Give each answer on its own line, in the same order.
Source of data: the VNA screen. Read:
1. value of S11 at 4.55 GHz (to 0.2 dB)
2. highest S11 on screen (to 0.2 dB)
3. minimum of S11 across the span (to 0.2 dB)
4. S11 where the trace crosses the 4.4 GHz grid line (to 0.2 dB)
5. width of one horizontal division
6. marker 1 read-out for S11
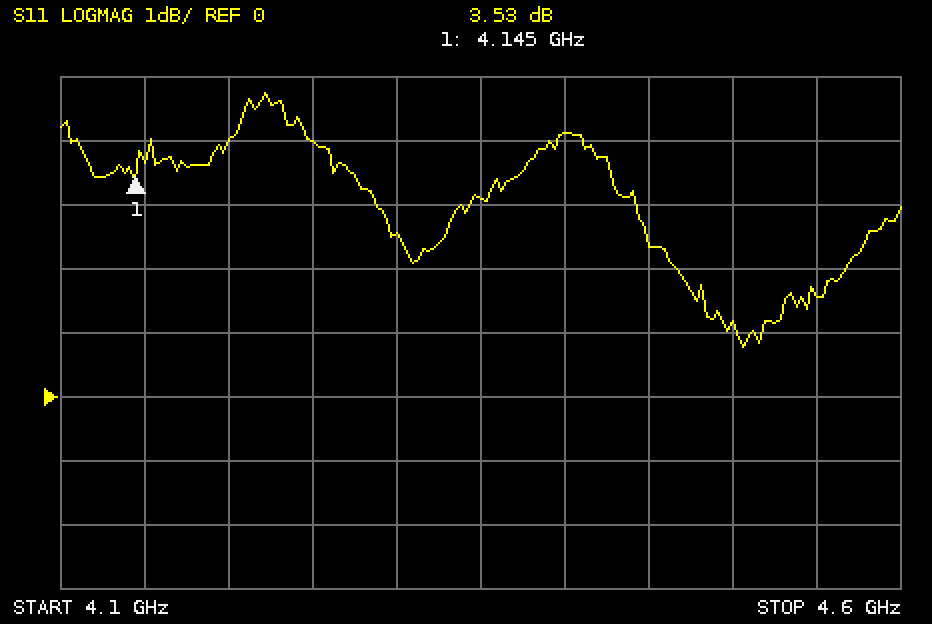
1.6 dB
4.8 dB
0.8 dB
4.2 dB
50 MHz
3.53 dB
